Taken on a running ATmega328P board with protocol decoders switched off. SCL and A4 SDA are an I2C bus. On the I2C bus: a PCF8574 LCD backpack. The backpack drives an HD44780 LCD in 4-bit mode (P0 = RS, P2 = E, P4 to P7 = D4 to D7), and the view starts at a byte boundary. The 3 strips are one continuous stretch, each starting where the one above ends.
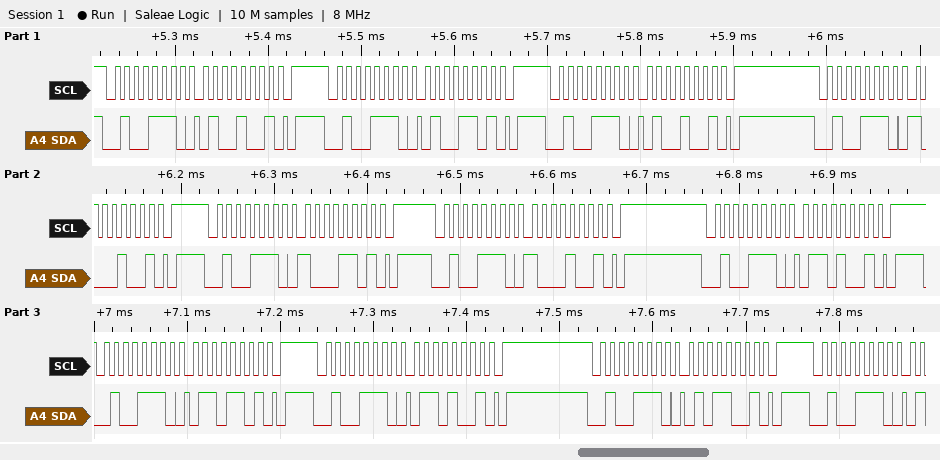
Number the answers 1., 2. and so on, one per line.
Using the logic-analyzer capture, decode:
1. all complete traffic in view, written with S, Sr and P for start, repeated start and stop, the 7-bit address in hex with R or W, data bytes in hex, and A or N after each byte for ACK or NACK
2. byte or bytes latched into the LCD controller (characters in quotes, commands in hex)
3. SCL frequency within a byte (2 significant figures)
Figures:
1. S 27W A 49 A P S 27W A 4D A P S 27W A 49 A P S 27W A 89 A P S 27W A 8D A P S 27W A 89 A P S 27W A 69 A P S 27W A 6D A P S 27W A 69 A P S 27W A 59 A P S 27W A
2. 'H'
3. 100 kHz
